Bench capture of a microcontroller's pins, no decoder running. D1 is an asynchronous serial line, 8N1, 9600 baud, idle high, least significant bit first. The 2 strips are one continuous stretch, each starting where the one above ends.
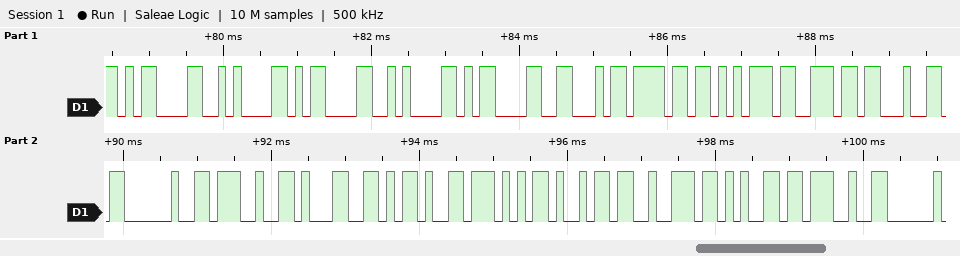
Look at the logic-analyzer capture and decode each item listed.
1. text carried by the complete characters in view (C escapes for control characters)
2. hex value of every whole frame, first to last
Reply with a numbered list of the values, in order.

1. "\r\n\r\n\rFound '1-Wire'"
2. 0D 0A 0D 0A 0D 46 6F 75 6E 64 20 27 31 2D 57 69 72 65 27
